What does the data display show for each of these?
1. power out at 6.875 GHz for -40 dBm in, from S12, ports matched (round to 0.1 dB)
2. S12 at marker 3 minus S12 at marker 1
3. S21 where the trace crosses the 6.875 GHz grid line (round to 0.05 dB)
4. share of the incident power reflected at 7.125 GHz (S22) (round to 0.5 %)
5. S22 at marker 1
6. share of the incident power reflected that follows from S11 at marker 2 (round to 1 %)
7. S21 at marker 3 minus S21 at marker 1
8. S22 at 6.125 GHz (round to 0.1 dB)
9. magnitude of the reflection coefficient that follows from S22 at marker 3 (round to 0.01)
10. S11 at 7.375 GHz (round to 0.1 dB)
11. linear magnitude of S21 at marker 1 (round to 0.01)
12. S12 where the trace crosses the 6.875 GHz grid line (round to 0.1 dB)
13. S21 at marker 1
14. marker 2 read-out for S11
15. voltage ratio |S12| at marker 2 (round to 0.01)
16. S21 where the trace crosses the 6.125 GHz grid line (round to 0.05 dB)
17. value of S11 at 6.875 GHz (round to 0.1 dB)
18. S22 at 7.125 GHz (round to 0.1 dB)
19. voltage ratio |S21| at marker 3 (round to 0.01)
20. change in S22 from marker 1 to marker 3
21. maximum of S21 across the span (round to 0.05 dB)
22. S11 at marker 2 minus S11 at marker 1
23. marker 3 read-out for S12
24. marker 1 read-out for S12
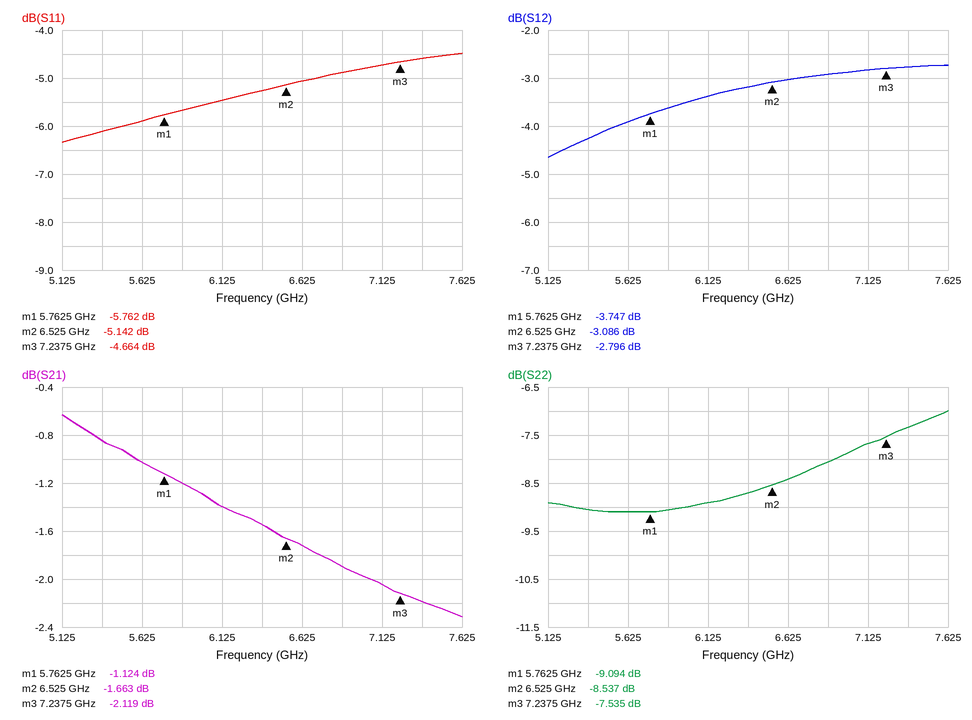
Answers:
-42.9 dBm
0.951 dB
-1.90 dB
17.0 %
-9.094 dB
31 %
-0.995 dB
-8.9 dB
0.42
-4.6 dB
0.88
-2.9 dB
-1.124 dB
-5.142 dB
0.70
-1.40 dB
-4.9 dB
-7.7 dB
0.78
1.559 dB
-0.65 dB
0.620 dB
-2.796 dB
-3.747 dB
